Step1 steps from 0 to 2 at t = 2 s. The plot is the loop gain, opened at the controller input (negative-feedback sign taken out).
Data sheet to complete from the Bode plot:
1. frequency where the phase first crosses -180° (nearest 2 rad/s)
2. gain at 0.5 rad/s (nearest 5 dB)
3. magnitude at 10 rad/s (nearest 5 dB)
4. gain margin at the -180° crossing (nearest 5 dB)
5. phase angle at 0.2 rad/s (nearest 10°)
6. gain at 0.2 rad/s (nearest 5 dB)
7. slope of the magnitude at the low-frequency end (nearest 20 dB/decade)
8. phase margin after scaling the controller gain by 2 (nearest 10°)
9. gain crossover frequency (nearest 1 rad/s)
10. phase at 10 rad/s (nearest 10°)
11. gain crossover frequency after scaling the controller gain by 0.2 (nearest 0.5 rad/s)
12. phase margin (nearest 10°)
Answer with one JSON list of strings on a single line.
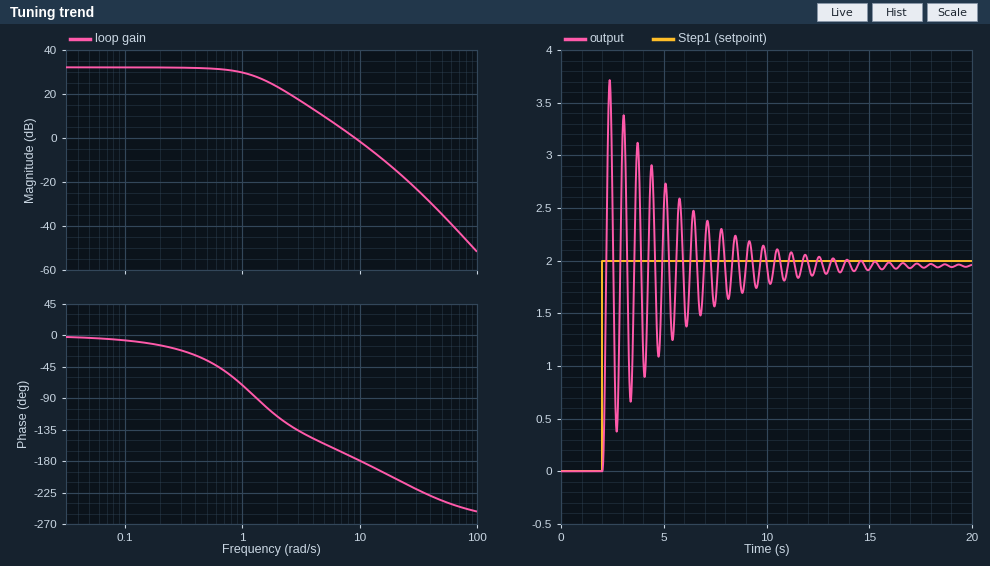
["10 rad/s", "30 dB", "0 dB", "0 dB", "-10°", "30 dB", "0 dB/decade", "-10°", "9 rad/s", "-180°", "4.0 rad/s", "0°"]
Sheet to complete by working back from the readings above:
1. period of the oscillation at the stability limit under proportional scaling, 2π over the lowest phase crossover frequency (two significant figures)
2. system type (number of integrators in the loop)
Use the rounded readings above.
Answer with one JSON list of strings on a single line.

["0.63 s", "0"]
